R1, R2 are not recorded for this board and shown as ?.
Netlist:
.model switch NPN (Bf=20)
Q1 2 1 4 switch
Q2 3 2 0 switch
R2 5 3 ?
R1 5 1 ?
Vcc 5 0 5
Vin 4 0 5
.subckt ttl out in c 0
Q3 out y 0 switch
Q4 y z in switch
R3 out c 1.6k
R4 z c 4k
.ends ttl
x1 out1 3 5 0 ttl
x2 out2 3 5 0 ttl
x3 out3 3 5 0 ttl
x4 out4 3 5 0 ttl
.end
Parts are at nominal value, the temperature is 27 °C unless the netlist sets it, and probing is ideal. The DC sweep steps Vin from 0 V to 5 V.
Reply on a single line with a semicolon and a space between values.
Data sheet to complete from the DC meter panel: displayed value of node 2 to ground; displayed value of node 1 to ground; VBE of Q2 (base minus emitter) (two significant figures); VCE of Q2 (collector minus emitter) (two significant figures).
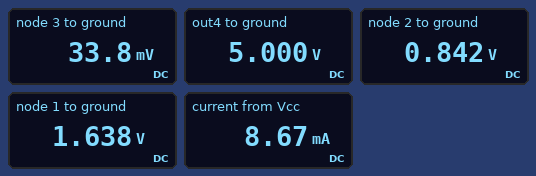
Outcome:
0.842 V; 1.638 V; 840 mV; 34 mV
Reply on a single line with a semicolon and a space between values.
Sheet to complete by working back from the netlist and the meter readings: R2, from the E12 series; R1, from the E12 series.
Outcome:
2.2 kΩ; 1.5 kΩ
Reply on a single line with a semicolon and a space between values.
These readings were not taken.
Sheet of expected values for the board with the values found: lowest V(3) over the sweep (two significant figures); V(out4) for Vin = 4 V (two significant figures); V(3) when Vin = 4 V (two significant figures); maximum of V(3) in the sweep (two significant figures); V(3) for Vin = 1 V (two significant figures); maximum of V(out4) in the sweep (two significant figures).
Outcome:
34 mV; 5.0 V; 34 mV; 840 mV; 34 mV; 5.0 V
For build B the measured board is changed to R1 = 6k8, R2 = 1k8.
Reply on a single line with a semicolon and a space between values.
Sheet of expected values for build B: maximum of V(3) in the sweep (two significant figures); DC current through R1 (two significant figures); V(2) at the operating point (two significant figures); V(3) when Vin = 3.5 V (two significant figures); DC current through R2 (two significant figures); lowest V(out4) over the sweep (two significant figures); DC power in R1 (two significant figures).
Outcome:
850 mV; 500 µA; 830 mV; 67 mV; 2.7 mA; 40 mV; 1.7 mW
